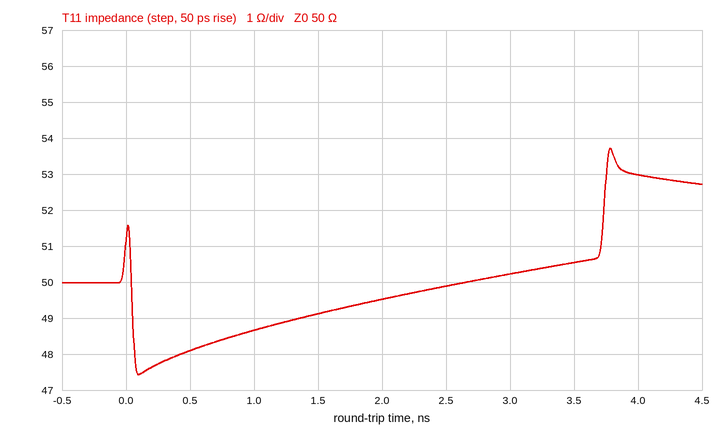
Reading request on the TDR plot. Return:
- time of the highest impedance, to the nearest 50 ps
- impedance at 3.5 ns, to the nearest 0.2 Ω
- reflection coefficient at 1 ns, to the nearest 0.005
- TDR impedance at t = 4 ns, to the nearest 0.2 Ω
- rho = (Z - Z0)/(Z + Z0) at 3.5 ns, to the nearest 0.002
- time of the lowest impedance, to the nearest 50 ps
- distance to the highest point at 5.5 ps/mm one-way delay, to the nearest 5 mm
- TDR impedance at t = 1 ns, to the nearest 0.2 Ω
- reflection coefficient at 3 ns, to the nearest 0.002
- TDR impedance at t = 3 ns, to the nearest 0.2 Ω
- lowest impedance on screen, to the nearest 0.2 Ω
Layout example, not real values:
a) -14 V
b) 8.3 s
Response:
a) 3.80 ns
b) 50.6 Ω
c) -0.015
d) 53.0 Ω
e) +0.006
f) 100 ps
g) 345 mm
h) 48.6 Ω
i) +0.002
j) 50.2 Ω
k) 47.4 Ω
